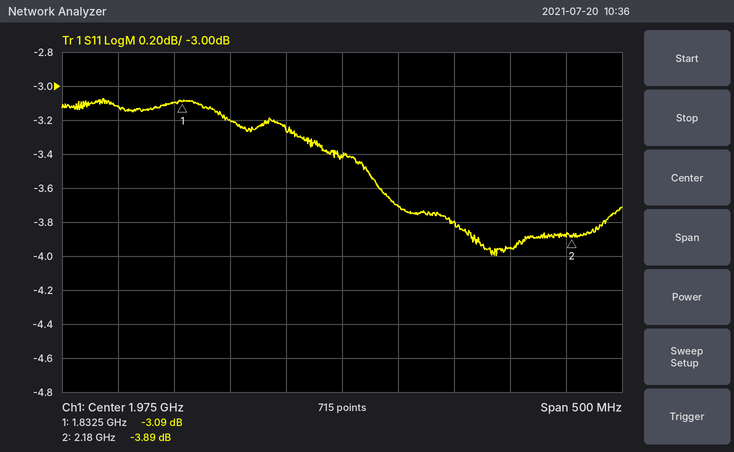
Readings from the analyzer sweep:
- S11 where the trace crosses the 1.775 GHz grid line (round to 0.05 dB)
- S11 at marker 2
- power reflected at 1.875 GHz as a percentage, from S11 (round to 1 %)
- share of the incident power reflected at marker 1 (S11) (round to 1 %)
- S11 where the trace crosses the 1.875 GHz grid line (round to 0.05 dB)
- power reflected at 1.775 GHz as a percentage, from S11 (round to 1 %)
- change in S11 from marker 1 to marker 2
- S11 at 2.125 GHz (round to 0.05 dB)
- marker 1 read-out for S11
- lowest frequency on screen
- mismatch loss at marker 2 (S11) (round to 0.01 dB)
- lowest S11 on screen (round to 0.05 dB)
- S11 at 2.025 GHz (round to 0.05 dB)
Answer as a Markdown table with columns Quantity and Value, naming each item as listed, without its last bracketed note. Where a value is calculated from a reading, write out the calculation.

| Quantity | Value |
|---|---|
| S11 where the trace crosses the 1.775 GHz grid line | -3.10 dB |
| S11 at marker 2 | -3.89 dB |
| power reflected at 1.875 GHz as a percentage, from S11 | 10^(-3.2/10) ≈ 48 % |
| share of the incident power reflected at marker 1 (S11) | 10^(-3.09/10) ≈ 49 % |
| S11 where the trace crosses the 1.875 GHz grid line | -3.20 dB |
| power reflected at 1.775 GHz as a percentage, from S11 | 10^(-3.1/10) ≈ 49 % |
| change in S11 from marker 1 to marker 2 | -3.89 − (-3.09) = -0.80 dB |
| S11 at 2.125 GHz | -3.95 dB |
| marker 1 read-out for S11 | -3.09 dB |
| lowest frequency on screen | 1.725 GHz |
| mismatch loss at marker 2 (S11) | −10 log10(1 − 10^(-3.89/10)) ≈ 2.28 dB |
| lowest S11 on screen | -4.00 dB |
| S11 at 2.025 GHz | -3.70 dB |
